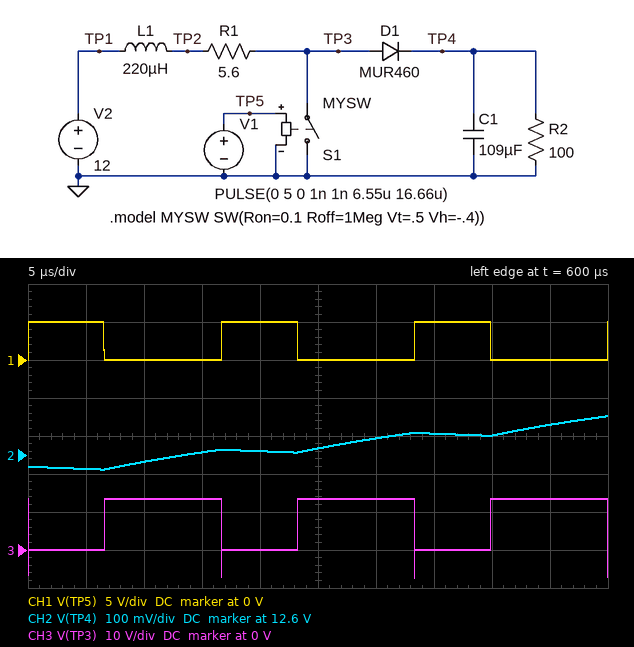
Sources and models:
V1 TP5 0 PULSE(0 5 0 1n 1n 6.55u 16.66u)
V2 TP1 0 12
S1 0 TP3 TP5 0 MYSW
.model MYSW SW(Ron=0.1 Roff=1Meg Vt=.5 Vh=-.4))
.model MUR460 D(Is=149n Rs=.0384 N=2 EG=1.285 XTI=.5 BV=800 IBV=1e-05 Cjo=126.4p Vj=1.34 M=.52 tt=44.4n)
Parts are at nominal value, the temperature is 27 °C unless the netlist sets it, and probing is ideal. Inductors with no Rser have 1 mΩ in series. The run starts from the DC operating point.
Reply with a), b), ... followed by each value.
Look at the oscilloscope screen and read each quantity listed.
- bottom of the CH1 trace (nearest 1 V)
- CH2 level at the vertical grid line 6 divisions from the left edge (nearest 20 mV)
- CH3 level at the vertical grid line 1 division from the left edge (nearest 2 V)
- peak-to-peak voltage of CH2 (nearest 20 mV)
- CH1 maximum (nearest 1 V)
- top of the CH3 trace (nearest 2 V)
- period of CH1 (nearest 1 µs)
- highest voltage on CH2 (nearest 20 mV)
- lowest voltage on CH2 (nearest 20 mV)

a) 0 V
b) 12.64 V
c) 0 V
d) 140 mV
e) 5 V
f) 14 V
g) 17 µs
h) 12.70 V
i) 12.56 V
